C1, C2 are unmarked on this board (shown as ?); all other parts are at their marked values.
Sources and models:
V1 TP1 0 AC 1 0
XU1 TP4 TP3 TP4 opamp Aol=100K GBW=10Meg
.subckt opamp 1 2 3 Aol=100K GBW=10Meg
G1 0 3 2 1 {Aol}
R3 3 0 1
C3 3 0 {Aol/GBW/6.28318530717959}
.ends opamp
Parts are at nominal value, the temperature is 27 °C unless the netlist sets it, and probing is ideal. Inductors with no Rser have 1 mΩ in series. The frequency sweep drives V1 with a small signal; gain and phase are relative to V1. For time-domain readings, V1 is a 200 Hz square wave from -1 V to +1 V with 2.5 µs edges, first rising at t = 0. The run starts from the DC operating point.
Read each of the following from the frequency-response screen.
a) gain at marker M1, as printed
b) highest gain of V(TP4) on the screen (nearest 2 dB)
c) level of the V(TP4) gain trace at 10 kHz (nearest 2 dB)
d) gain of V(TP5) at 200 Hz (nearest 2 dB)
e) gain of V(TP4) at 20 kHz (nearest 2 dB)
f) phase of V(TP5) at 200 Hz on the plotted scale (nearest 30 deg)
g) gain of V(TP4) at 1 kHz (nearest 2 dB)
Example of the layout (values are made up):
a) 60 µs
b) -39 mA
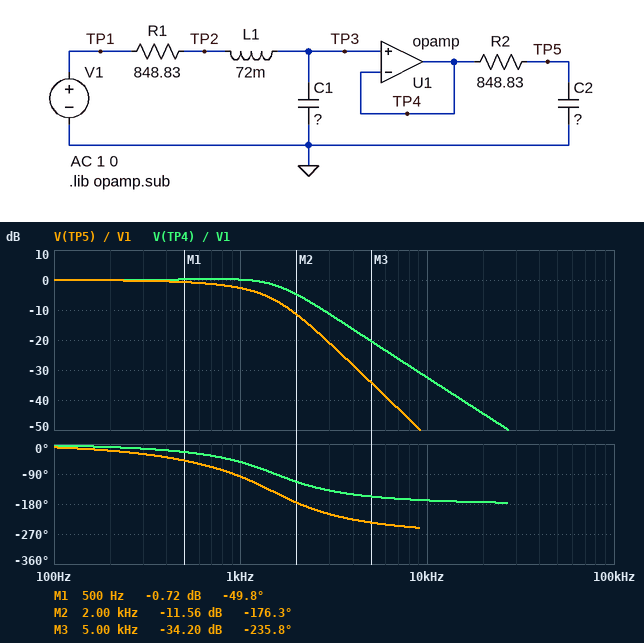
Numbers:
a) -0.72 dB
b) 0 dB
c) -32 dB
d) 0 dB
e) -44 dB
f) -30 deg
g) 0 dB
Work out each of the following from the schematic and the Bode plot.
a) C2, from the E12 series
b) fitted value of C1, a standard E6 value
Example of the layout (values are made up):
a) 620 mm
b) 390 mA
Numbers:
a) 180 nF
b) 150 nF
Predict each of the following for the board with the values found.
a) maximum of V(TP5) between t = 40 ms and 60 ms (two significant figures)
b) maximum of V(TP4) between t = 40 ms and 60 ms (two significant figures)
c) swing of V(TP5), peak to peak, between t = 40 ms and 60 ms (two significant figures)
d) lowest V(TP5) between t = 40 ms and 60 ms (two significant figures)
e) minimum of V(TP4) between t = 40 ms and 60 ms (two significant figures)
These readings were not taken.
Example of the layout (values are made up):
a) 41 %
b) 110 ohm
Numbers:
a) 1.0 V
b) 1.2 V
c) 2.0 V
d) -1.0 V
e) -1.2 V
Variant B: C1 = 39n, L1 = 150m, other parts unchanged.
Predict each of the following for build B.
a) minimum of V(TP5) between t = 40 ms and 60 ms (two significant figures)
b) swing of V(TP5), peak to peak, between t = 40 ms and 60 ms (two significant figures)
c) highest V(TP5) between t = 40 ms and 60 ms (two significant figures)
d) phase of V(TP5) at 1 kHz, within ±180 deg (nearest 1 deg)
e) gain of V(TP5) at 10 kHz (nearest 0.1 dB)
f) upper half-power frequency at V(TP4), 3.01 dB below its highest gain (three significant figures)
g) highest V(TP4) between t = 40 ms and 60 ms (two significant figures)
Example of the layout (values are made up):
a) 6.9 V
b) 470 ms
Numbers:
a) -1.2 V
b) 2.4 V
c) 1.2 V
d) -59 deg
e) -46.6 dB
f) 2.40 kHz
g) 2.0 V
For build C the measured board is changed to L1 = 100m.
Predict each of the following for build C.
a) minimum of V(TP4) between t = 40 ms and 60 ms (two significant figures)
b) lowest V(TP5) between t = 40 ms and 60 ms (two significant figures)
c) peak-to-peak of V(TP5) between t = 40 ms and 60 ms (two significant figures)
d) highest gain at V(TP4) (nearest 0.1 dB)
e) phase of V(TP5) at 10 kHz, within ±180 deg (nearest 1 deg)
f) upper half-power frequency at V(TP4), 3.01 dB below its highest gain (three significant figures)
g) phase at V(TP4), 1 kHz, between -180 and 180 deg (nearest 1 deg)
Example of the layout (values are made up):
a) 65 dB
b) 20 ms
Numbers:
a) -1.3 V
b) -1.1 V
c) 2.2 V
d) 1.0 dB
e) 104 deg
f) 1.51 kHz
g) -63 deg
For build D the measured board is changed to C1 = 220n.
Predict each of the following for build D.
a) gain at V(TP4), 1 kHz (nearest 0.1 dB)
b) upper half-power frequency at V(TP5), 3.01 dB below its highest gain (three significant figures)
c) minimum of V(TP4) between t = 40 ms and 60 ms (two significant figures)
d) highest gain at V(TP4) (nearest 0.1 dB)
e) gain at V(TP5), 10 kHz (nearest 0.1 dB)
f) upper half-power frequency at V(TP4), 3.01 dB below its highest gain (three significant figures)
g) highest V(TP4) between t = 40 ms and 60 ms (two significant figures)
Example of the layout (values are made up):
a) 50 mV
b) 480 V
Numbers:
a) -1.8 dB
b) 808 Hz
c) -1.1 V
d) 0 dB
e) -55.6 dB
f) 1.20 kHz
g) 1.1 V
